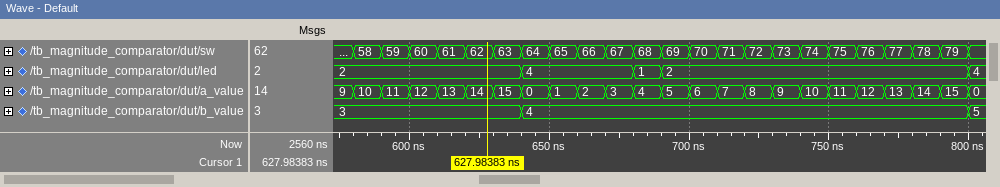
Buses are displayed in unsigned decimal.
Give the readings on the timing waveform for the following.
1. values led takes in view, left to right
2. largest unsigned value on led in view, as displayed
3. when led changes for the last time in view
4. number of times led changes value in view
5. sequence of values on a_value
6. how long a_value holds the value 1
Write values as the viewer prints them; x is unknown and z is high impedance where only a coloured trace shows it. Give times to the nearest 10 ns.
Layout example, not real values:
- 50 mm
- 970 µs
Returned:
- 2, 4, 1, 2, 4
- 4
- 800 ns
- 4
- 9, 10, 11, 12, 13, 14, 15, 0, 1, 2, 3, 4, 5, 6, 7, 8, 9, 10, 11, 12, 13, 14, 15, 0
- 10 ns
